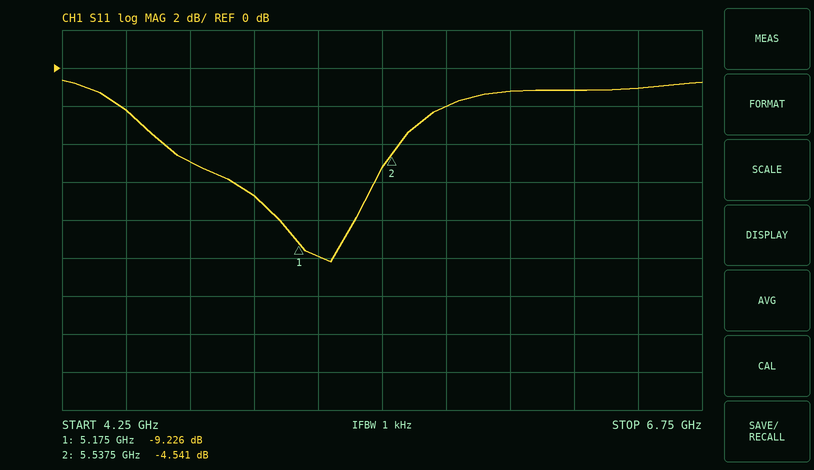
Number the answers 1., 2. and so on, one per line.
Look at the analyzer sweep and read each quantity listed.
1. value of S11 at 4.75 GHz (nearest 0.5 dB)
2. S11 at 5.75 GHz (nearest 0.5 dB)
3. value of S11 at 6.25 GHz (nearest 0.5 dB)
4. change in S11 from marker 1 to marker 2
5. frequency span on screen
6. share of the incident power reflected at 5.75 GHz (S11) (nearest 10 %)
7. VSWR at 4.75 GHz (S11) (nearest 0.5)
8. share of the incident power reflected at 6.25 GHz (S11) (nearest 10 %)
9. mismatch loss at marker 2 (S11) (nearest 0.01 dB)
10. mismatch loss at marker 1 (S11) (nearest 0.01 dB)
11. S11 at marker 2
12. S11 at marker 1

1. -5.0 dB
2. -2.0 dB
3. -1.0 dB
4. 4.685 dB
5. 2.5 GHz
6. 60 %
7. 3.5
8. 80 %
9. 1.88 dB
10. 0.55 dB
11. -4.541 dB
12. -9.226 dB
